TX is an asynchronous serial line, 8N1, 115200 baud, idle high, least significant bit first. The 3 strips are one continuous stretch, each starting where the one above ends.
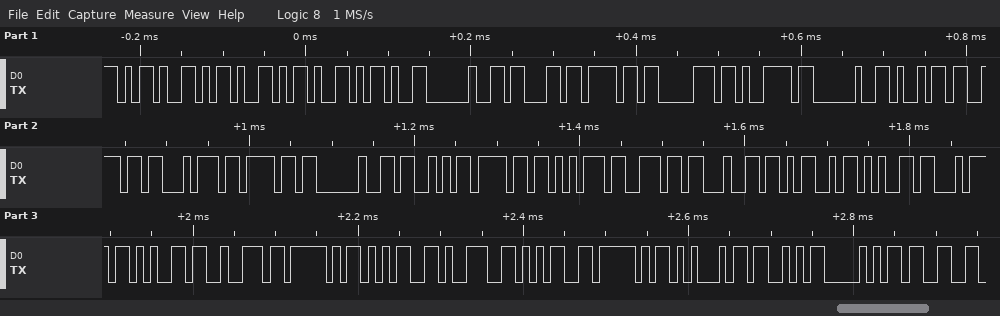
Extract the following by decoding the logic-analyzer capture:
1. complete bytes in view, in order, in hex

2D 2D 2D 2D 20 63 6F 70 79 20 69 6E 74 6F 20 53 6F 75 6E 64 4D 65 74 65 72 5F 35 39 35 5F 45 53 50 33
